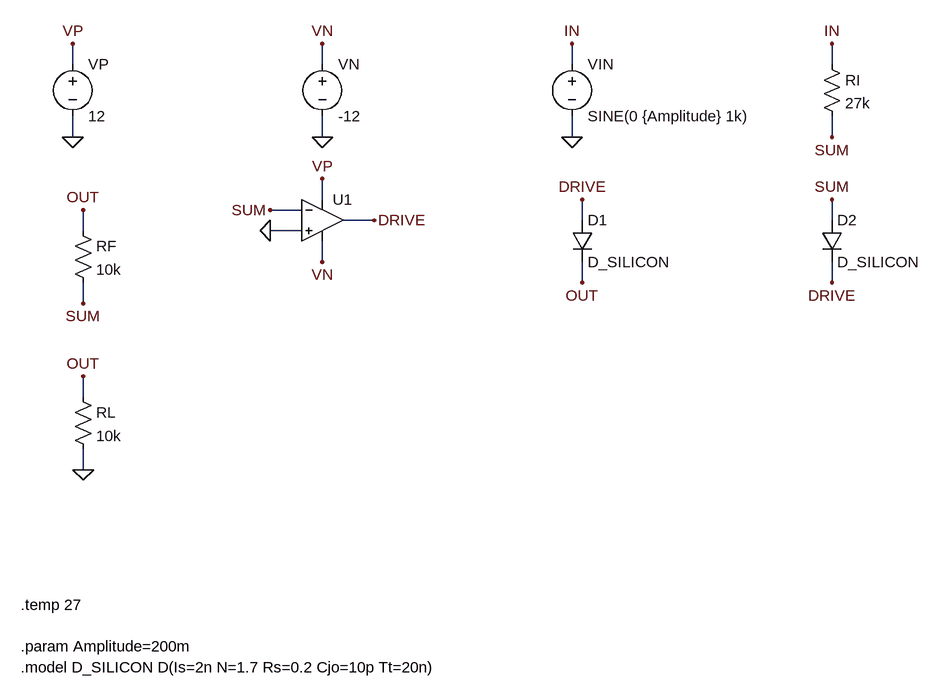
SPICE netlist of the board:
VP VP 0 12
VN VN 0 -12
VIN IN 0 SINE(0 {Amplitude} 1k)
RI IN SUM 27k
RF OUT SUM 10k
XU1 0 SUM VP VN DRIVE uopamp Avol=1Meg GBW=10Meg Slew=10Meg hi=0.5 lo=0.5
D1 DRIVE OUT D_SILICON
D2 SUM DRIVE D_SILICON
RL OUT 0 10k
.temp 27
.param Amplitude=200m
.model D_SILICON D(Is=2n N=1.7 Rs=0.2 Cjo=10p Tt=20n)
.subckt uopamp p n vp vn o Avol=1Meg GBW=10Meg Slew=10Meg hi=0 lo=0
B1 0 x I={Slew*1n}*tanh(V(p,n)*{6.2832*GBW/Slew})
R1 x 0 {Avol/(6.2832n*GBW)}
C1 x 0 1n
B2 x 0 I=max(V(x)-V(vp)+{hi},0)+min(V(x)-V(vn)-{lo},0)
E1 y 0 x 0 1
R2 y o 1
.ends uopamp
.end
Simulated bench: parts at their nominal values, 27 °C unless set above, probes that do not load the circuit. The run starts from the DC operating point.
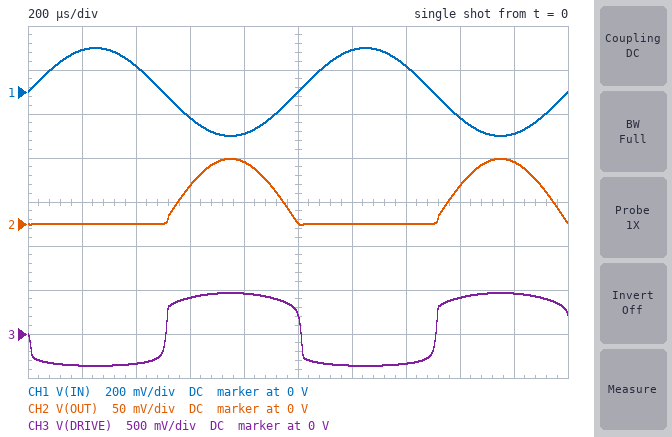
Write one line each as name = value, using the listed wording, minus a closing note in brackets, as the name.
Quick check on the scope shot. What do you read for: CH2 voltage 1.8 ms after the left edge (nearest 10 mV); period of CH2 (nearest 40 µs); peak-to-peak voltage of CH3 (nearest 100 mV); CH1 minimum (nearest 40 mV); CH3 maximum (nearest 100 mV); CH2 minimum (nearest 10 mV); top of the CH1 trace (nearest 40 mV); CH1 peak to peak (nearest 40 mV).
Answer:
CH2 voltage 1.8 ms after the left edge = 70 mV
period of CH2 = 1.00 ms
peak-to-peak voltage of CH3 = 800 mV
CH1 minimum = -200 mV
CH3 maximum = 500 mV
CH2 minimum = 0 V
top of the CH1 trace = 200 mV
CH1 peak to peak = 400 mV
